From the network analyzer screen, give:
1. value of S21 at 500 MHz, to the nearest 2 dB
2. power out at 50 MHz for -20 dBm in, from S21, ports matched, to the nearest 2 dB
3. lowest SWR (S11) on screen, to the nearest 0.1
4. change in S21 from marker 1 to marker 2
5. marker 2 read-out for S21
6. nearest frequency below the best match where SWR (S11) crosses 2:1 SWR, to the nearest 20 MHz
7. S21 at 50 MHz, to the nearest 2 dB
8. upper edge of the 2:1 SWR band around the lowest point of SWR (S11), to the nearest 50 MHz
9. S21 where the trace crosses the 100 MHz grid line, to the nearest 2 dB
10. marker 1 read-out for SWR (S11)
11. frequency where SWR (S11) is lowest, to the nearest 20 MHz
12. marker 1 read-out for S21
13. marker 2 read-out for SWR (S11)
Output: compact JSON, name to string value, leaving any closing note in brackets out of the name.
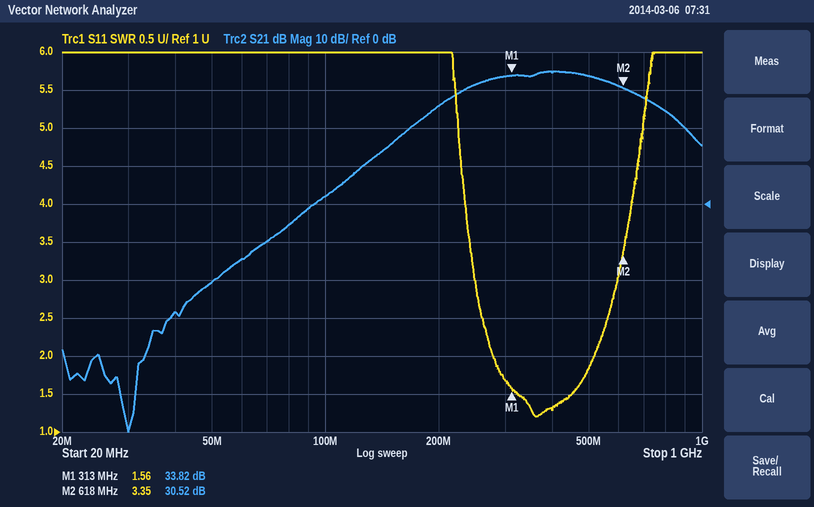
{"value of S21 at 500 MHz, to the nearest 2 dB": "34 dB", "power out at 50 MHz for -20 dBm in, from S21, ports matched, to the nearest 2 dB": "-40 dBm", "lowest SWR (S11) on screen, to the nearest 0.1": "1.2", "change in S21 from marker 1 to marker 2": "-3.30 dB", "marker 2 read-out for S21": "30.52 dB", "nearest frequency below the best match where SWR (S11) crosses 2:1 SWR, to the nearest 20 MHz": "280 MHz", "S21 at 50 MHz, to the nearest 2 dB": "-20 dB", "upper edge of the 2:1 SWR band around the lowest point of SWR (S11), to the nearest 50 MHz": "500 MHz", "S21 where the trace crosses the 100 MHz grid line, to the nearest 2 dB": "2 dB", "marker 1 read-out for SWR": "1.56", "frequency where SWR (S11) is lowest, to the nearest 20 MHz": "360 MHz", "marker 1 read-out for S21": "33.82 dB", "marker 2 read-out for SWR": "3.35"}
